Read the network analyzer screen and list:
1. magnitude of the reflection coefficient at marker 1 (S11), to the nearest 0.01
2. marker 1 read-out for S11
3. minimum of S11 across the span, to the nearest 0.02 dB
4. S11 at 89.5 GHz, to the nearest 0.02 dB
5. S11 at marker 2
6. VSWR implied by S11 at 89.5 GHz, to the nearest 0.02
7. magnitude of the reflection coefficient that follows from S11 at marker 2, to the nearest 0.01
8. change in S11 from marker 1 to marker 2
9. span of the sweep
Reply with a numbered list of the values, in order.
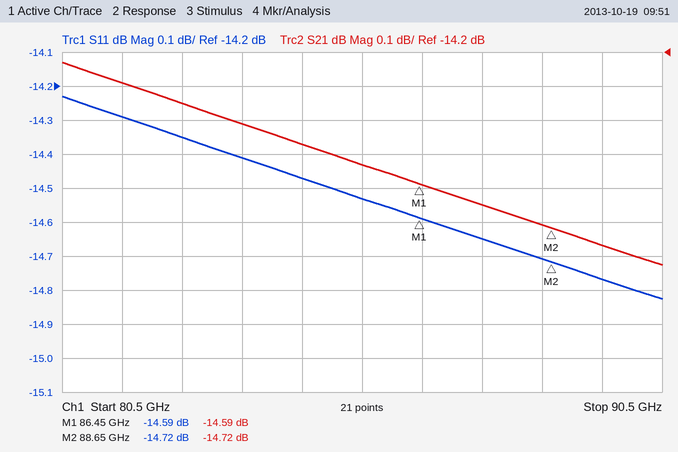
1. 0.19
2. -14.59 dB
3. -14.82 dB
4. -14.76 dB
5. -14.72 dB
6. 1.44
7. 0.18
8. -0.13 dB
9. 10 GHz
